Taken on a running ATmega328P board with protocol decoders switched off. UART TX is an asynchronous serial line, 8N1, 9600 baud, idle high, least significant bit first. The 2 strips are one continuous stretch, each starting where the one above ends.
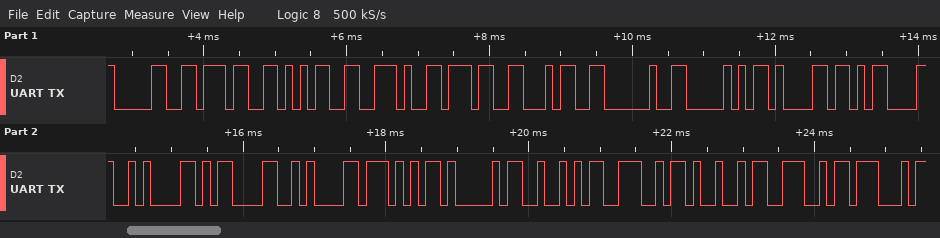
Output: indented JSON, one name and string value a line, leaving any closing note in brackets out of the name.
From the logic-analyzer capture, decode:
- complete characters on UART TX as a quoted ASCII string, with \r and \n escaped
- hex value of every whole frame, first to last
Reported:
{
  "complete characters on UART TX as a quoted ASCII string, with \\r and \\n escaped": "\"075.74 Pa\\r\\n\\r\\nWARNING\"",
  "hex value of every whole frame, first to last": "0x30 0x37 0x35 0x2E 0x37 0x34 0x20 0x50 0x61 0x0D 0x0A 0x0D 0x0A 0x57 0x41 0x52 0x4E 0x49 0x4E 0x47"
}
